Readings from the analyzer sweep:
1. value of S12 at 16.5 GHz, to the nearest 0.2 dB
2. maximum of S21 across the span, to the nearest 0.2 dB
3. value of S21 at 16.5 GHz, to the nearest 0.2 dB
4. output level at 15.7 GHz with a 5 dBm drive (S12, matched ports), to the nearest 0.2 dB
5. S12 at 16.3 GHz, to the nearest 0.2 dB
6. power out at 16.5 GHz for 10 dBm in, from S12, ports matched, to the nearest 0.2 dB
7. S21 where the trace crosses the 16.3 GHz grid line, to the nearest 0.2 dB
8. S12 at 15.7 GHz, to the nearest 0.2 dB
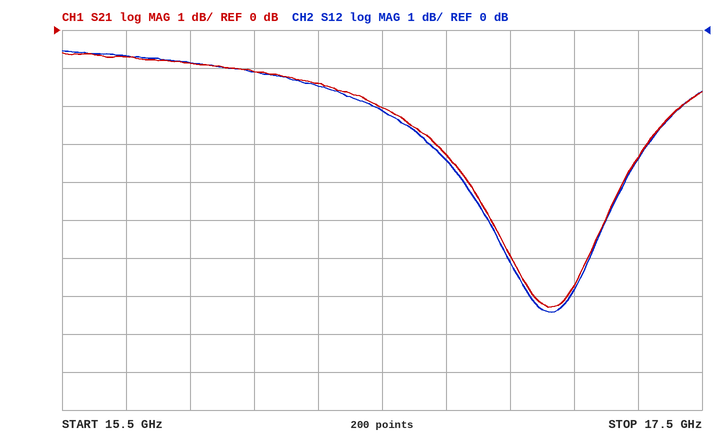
-2.2 dB
-0.6 dB
-2.0 dB
4.4 dBm
-1.4 dB
7.8 dBm
-1.4 dB
-0.6 dB
